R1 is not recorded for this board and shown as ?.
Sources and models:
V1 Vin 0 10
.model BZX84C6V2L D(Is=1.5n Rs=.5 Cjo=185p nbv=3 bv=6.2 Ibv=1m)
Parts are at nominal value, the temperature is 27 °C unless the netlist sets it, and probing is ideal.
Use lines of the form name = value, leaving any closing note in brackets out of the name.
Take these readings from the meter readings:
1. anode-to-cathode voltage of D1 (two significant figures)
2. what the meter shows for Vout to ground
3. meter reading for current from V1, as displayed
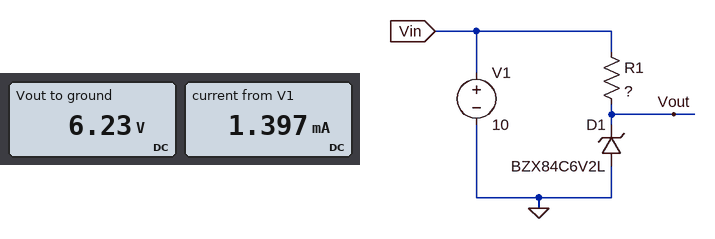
anode-to-cathode voltage of D1 = -6.2 V
what the meter shows for Vout to ground = 6.23 V
meter reading for current from V1, as displayed = 1.397 mA
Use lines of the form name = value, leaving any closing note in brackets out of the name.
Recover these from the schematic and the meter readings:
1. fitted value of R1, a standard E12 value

fitted value of R1, a standard E12 value = 2.7 kΩ
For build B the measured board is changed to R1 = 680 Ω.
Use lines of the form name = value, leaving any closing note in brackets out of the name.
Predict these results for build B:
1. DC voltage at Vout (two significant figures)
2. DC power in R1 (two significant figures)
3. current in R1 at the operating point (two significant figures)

DC voltage at Vout = 6.3 V
DC power in R1 = 20 mW
current in R1 at the operating point = 5.4 mA
